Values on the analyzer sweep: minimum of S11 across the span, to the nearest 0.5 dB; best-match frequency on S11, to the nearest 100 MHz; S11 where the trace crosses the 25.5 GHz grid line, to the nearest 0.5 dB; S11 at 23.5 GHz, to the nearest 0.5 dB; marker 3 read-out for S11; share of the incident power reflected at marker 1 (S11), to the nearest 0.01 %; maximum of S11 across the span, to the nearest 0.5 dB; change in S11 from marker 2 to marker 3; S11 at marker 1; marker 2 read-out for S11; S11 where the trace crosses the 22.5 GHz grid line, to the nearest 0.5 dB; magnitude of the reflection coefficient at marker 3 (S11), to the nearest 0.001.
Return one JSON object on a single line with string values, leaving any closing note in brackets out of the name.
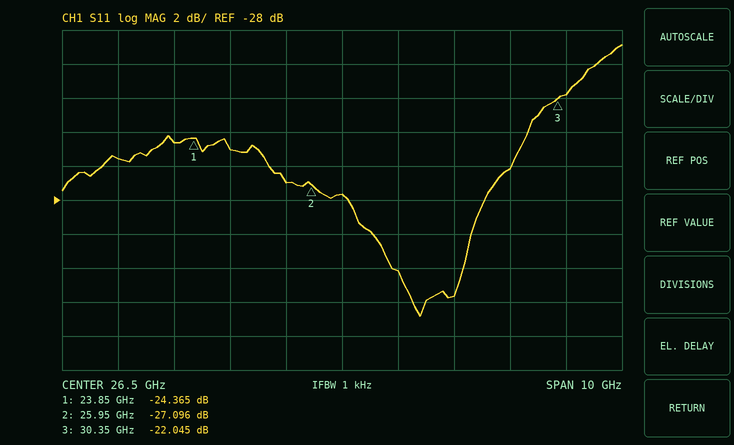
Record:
{"minimum of S11 across the span, to the nearest 0.5 dB": "-35.0 dB", "best-match frequency on S11, to the nearest 100 MHz": "27.9 GHz", "S11 where the trace crosses the 25.5 GHz grid line, to the nearest 0.5 dB": "-27.0 dB", "S11 at 23.5 GHz, to the nearest 0.5 dB": "-24.5 dB", "marker 3 read-out for S11": "-22.045 dB", "share of the incident power reflected at marker 1 (S11), to the nearest 0.01 %": "0.37 %", "maximum of S11 across the span, to the nearest 0.5 dB": "-19.0 dB", "change in S11 from marker 2 to marker 3": "5.051 dB", "S11 at marker 1": "-24.365 dB", "marker 2 read-out for S11": "-27.096 dB", "S11 where the trace crosses the 22.5 GHz grid line, to the nearest 0.5 dB": "-25.5 dB", "magnitude of the reflection coefficient at marker 3 (S11), to the nearest 0.001": "0.079"}
